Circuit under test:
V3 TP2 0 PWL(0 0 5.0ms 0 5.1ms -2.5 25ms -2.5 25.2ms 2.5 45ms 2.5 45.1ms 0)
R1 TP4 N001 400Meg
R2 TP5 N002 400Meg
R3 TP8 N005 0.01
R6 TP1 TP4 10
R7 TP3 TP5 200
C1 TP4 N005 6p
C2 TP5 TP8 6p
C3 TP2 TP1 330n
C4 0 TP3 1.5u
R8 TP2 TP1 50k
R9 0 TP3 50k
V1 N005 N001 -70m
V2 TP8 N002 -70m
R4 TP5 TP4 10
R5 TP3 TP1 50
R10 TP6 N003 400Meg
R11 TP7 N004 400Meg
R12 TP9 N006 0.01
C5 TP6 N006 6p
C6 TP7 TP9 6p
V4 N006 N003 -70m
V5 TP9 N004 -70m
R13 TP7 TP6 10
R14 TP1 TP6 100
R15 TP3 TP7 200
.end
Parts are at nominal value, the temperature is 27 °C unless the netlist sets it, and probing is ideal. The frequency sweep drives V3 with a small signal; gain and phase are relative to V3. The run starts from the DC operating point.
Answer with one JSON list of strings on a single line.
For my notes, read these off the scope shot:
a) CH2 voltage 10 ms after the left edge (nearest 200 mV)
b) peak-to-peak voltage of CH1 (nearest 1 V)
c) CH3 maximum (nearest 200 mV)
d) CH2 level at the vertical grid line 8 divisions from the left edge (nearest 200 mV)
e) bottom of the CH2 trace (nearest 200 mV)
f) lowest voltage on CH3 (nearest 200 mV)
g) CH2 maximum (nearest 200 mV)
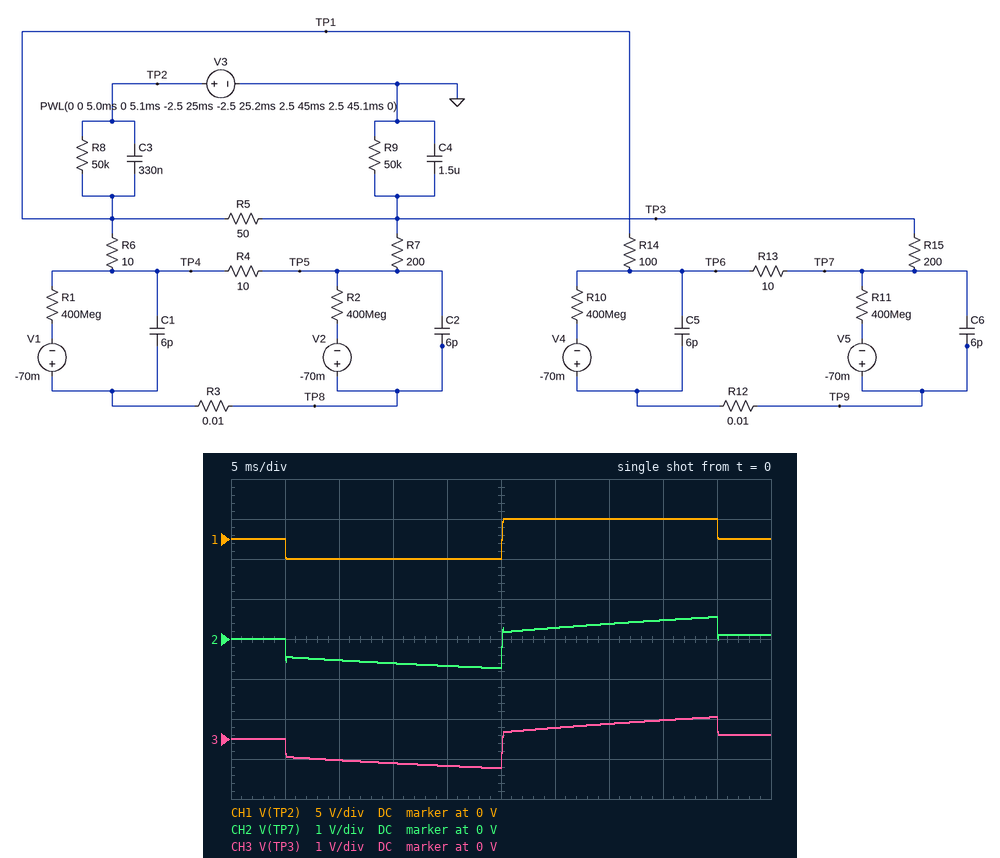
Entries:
["-600 mV", "5 V", "600 mV", "400 mV", "-800 mV", "-800 mV", "600 mV"]
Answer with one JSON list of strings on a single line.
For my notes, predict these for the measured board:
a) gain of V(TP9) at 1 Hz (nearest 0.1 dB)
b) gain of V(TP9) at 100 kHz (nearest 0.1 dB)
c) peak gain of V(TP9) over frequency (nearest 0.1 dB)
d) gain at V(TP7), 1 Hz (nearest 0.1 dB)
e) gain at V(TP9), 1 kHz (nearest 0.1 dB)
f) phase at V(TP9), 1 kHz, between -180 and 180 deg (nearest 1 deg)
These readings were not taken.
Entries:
["-6.3 dB", "-3.7 dB", "-3.6 dB", "-6.3 dB", "-14.7 dB", "9 deg"]
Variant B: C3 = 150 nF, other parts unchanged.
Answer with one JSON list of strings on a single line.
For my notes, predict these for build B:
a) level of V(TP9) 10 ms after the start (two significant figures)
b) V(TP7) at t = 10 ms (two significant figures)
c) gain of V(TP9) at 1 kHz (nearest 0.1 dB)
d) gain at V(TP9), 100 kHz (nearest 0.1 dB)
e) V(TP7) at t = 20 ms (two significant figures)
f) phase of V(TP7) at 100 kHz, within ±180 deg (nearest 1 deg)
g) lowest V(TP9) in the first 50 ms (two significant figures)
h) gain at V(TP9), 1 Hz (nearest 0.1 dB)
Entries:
["-410 mV", "-340 mV", "-20.6 dB", "-4.0 dB", "-540 mV", "15 deg", "-690 mV", "-6.3 dB"]
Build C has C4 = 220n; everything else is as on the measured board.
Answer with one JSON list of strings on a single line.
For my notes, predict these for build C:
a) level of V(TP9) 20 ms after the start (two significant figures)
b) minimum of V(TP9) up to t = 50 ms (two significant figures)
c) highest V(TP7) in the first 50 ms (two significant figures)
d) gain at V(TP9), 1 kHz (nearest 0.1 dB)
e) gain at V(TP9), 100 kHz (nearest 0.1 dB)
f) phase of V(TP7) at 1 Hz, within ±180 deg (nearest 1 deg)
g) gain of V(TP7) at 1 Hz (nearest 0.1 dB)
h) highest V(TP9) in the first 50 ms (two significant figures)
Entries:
["-1.4 V", "-1.6 V", "1.7 V", "-4.4 dB", "-3.7 dB", "1 deg", "-6.0 dB", "1.6 V"]
